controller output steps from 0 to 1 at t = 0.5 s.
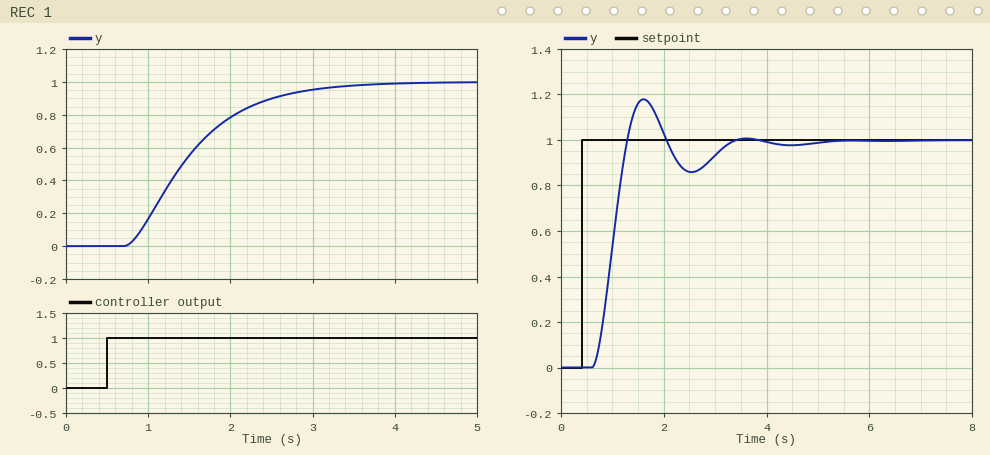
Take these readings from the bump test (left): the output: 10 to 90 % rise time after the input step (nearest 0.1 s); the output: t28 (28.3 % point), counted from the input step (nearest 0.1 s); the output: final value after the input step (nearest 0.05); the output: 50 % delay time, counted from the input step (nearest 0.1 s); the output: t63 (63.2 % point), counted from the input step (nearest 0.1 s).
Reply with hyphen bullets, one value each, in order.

- 1.6 s
- 0.6 s
- 1.00
- 0.9 s
- 1.1 s
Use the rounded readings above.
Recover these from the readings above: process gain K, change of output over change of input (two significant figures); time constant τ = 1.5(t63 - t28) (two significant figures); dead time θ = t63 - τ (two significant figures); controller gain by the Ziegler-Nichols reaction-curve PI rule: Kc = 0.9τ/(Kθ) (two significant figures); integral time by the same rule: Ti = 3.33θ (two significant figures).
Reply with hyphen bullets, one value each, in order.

- 1.0
- 0.75 s
- 0.35 s
- 1.9
- 1.2 s
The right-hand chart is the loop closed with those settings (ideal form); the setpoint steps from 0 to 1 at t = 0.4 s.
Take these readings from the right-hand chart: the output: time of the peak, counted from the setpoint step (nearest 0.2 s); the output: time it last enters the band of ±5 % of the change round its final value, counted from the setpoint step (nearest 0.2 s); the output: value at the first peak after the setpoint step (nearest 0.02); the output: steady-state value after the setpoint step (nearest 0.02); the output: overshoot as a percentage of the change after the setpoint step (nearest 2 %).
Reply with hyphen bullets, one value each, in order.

- 1.2 s
- 2.6 s
- 1.18
- 1.00
- 18 %
